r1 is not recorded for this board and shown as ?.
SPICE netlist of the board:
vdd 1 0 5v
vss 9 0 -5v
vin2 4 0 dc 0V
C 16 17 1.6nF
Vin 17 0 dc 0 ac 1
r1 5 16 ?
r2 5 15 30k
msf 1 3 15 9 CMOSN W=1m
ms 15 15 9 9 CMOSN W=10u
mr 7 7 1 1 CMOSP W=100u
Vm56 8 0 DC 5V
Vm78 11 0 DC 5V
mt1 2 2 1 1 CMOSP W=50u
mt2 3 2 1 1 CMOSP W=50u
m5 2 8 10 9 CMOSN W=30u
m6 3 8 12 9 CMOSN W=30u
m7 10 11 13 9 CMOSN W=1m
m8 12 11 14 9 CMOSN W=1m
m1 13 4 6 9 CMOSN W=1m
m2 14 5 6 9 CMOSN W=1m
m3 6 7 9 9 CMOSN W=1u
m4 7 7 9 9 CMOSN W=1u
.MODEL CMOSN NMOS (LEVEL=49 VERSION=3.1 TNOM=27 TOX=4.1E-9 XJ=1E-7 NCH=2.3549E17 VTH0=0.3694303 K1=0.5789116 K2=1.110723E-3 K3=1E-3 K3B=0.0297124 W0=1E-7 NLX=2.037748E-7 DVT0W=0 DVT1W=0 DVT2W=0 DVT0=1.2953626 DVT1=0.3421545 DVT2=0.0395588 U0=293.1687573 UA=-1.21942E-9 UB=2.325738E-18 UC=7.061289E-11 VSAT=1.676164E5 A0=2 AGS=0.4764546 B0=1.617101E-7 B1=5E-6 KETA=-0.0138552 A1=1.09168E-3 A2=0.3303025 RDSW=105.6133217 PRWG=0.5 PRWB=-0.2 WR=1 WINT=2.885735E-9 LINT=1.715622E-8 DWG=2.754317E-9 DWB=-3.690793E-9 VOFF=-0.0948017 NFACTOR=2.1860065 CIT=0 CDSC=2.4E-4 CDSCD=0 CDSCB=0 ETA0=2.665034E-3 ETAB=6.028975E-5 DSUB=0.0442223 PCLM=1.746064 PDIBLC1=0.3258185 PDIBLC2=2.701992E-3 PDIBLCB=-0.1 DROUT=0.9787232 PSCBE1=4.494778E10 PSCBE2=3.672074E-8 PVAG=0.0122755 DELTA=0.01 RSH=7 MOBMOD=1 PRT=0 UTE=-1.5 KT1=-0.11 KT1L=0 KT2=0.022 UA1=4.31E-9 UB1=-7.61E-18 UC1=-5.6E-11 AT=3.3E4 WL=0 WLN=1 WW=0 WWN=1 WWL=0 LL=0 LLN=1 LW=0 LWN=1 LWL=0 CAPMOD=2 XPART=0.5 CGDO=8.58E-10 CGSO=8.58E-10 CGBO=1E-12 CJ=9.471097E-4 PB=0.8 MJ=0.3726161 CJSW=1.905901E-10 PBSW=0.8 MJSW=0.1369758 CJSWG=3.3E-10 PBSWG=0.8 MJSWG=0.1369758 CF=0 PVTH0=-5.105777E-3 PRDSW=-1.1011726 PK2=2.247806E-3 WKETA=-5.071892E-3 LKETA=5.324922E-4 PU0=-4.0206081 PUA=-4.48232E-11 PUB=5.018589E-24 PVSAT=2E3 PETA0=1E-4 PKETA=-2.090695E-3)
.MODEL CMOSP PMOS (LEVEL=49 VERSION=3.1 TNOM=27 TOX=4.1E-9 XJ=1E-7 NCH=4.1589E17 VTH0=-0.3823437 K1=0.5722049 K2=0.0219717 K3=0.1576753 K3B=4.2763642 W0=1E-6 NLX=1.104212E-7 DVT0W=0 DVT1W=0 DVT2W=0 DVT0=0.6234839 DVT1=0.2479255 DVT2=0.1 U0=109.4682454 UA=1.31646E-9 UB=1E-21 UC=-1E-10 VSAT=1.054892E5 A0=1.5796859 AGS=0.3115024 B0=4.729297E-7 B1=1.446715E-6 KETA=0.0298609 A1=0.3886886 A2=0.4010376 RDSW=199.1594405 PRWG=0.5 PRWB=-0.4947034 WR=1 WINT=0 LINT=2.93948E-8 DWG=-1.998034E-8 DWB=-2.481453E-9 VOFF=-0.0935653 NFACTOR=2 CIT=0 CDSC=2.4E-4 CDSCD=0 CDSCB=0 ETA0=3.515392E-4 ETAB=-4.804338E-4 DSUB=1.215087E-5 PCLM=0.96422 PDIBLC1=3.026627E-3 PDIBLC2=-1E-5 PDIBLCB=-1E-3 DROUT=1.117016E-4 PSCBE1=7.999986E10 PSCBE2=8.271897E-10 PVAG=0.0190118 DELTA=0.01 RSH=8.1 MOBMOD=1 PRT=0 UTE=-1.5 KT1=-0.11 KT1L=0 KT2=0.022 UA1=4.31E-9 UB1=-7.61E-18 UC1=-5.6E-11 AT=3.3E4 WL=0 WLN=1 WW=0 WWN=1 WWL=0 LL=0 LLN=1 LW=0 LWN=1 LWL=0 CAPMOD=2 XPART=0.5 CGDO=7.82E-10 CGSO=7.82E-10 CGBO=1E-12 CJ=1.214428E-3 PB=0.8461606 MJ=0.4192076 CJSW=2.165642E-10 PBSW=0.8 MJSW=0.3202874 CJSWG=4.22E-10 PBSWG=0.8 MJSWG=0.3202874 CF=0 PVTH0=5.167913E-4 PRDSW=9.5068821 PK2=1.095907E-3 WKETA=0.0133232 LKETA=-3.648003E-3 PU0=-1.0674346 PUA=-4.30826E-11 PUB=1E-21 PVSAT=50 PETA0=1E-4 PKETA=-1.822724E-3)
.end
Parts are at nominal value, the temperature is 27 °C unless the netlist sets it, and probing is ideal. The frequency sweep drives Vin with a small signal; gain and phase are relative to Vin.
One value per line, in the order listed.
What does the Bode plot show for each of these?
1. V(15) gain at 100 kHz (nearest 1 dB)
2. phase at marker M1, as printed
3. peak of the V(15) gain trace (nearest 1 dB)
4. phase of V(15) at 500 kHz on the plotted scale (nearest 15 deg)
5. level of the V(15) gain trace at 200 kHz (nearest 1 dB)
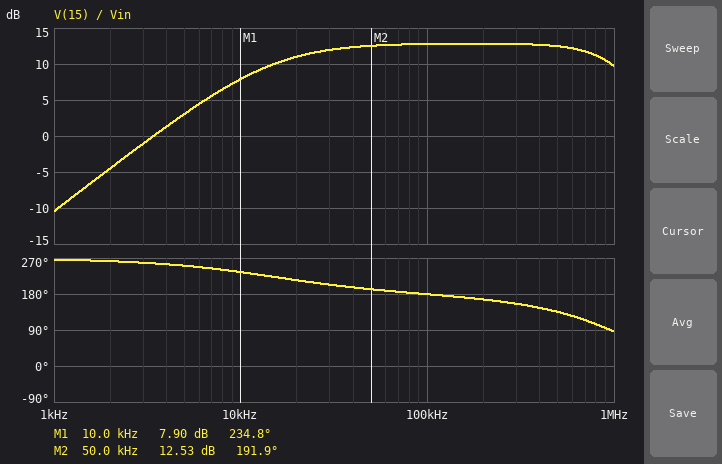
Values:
13 dB
234.8 deg
13 dB
135 deg
13 dB
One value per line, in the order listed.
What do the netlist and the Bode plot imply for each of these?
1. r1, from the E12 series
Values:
6.8 kΩ
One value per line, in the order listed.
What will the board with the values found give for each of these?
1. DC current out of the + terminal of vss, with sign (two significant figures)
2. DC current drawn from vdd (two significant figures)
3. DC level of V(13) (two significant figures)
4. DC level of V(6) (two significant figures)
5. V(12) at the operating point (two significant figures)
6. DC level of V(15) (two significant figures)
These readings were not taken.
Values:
-3.0 mA
3.0 mA
3.1 V
-1.1 V
1.5 V
4.7 mV
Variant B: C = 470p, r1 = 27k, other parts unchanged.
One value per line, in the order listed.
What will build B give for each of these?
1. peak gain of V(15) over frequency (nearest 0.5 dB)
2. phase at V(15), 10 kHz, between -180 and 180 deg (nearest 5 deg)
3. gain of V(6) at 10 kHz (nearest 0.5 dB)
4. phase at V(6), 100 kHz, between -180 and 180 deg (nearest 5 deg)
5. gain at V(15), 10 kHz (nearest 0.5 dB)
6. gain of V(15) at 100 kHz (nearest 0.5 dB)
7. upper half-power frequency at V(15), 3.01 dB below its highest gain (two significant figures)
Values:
6.0 dB
-130 deg
-62.0 dB
95 deg
-3.0 dB
1.0 dB
1.3 MHz
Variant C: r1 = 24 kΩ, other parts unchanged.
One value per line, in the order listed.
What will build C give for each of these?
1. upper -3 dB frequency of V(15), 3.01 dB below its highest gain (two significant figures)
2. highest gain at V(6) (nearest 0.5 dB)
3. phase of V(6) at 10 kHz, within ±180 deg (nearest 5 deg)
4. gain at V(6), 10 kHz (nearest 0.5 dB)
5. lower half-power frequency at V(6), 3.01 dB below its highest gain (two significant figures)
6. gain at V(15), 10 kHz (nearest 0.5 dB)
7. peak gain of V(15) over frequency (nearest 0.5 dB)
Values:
1.3 MHz
-11.0 dB
95 deg
-57.5 dB
870 kHz
1.0 dB
6.5 dB
